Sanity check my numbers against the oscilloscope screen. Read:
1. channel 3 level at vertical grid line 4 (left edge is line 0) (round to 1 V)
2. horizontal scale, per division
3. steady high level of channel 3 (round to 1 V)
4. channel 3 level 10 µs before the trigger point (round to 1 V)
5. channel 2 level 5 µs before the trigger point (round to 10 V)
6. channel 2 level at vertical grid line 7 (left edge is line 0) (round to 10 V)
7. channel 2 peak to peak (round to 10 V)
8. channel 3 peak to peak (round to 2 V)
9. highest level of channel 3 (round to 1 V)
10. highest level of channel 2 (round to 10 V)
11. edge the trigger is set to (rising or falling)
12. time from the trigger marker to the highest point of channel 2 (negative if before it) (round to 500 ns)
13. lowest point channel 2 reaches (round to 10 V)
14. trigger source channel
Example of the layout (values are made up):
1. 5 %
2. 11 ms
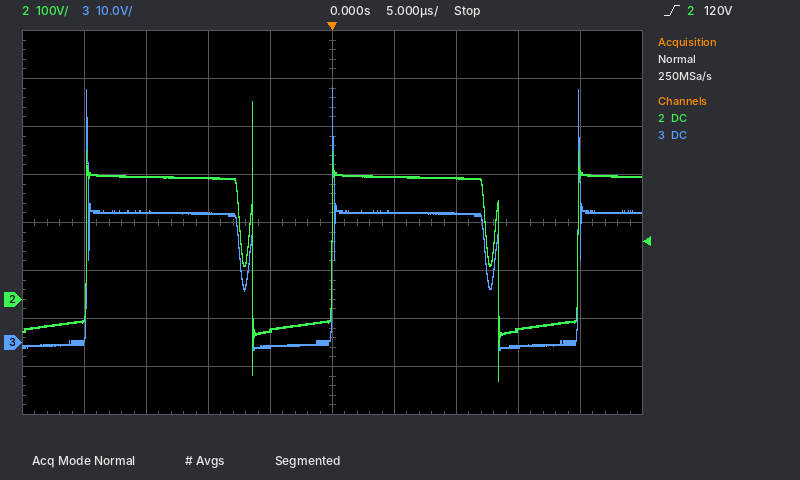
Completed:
1. -1 V
2. 5 µs
3. 27 V
4. 27 V
5. -60 V
6. 250 V
7. 580 V
8. 54 V
9. 53 V
10. 410 V
11. rising
12. -6.5 µs
13. -170 V
14. channel 2
